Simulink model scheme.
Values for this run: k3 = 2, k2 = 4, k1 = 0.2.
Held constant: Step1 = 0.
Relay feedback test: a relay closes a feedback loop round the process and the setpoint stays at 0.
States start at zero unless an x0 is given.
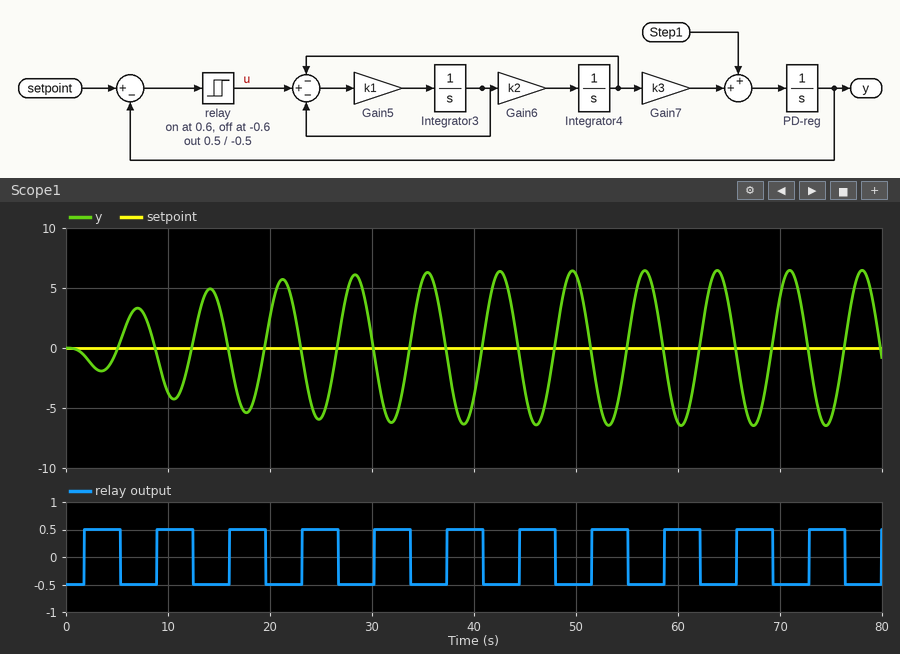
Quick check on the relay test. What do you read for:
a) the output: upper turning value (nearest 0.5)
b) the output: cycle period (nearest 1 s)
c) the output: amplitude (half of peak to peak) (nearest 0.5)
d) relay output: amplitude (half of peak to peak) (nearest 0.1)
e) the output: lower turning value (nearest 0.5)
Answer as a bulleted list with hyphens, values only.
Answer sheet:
- 6.5
- 7 s
- 6.5
- 0.5
- -6.5
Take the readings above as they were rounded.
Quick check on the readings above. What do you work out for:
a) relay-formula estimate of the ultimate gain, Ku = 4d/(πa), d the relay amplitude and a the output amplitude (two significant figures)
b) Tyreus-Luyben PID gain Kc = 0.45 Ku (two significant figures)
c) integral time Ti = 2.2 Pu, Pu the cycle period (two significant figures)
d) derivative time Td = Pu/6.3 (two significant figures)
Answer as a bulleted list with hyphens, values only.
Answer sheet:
- 0.098
- 0.044
- 15 s
- 1.1 s
